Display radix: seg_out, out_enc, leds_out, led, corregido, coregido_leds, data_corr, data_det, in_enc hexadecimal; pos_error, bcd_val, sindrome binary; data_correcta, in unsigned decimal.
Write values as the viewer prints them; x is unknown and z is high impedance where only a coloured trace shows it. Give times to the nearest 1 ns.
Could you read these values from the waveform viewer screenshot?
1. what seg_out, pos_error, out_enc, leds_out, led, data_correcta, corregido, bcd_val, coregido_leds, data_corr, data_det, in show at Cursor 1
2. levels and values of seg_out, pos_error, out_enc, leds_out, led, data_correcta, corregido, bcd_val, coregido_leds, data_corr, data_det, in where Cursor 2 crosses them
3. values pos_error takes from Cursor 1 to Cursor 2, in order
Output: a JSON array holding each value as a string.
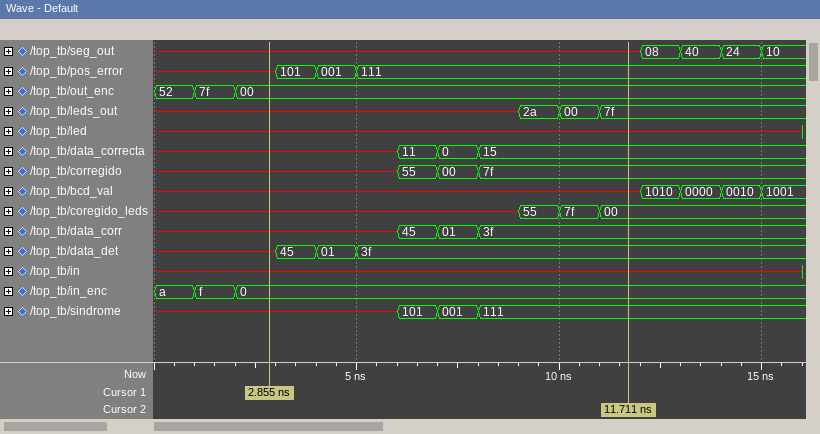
["seg_out=x, pos_error=x, out_enc=00, leds_out=x, led=x, data_correcta=x, corregido=x, bcd_val=x, coregido_leds=x, data_corr=x, data_det=x, in=x", "seg_out=x, pos_error=111, out_enc=00, leds_out=7f, led=x, data_correcta=15, corregido=7f, bcd_val=x, coregido_leds=00, data_corr=3f, data_det=3f, in=x", "x, 101, 001, 111"]
